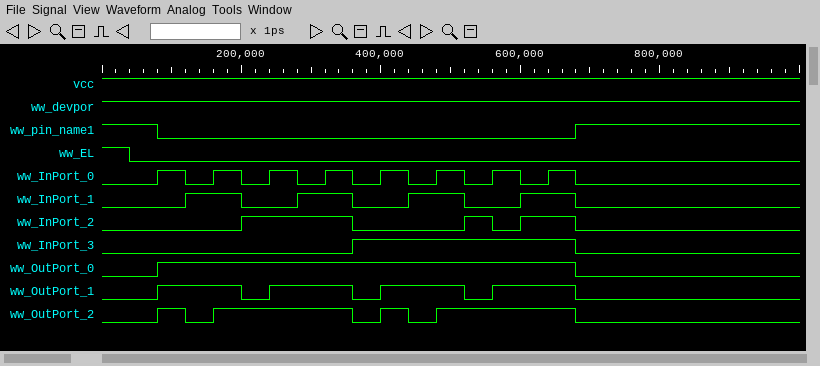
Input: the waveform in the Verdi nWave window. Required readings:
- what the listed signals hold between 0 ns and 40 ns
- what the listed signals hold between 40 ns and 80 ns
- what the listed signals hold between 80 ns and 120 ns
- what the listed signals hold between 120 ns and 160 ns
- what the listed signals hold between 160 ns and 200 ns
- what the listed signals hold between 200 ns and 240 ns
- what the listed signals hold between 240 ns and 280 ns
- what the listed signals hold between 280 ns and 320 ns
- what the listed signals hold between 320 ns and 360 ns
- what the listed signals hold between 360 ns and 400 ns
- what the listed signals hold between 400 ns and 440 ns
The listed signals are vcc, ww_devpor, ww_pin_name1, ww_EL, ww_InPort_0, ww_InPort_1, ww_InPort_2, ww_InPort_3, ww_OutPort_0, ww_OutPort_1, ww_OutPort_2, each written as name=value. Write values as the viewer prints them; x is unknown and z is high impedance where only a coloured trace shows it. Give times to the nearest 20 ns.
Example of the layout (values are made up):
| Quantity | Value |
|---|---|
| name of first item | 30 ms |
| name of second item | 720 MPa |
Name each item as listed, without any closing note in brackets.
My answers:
| Quantity | Value |
|---|---|
| what the listed signals hold between 0 ns and 40 ns | vcc=1, ww_devpor=1, ww_pin_name1=1, ww_EL=1, ww_InPort_0=0, ww_InPort_1=0, ww_InPort_2=0, ww_InPort_3=0, ww_OutPort_0=0, ww_OutPort_1=0, ww_OutPort_2=0 |
| what the listed signals hold between 40 ns and 80 ns | vcc=1, ww_devpor=1, ww_pin_name1=1, ww_EL=0, ww_InPort_0=0, ww_InPort_1=0, ww_InPort_2=0, ww_InPort_3=0, ww_OutPort_0=0, ww_OutPort_1=0, ww_OutPort_2=0 |
| what the listed signals hold between 80 ns and 120 ns | vcc=1, ww_devpor=1, ww_pin_name1=0, ww_EL=0, ww_InPort_0=1, ww_InPort_1=0, ww_InPort_2=0, ww_InPort_3=0, ww_OutPort_0=1, ww_OutPort_1=1, ww_OutPort_2=1 |
| what the listed signals hold between 120 ns and 160 ns | vcc=1, ww_devpor=1, ww_pin_name1=0, ww_EL=0, ww_InPort_0=0, ww_InPort_1=1, ww_InPort_2=0, ww_InPort_3=0, ww_OutPort_0=1, ww_OutPort_1=1, ww_OutPort_2=0 |
| what the listed signals hold between 160 ns and 200 ns | vcc=1, ww_devpor=1, ww_pin_name1=0, ww_EL=0, ww_InPort_0=1, ww_InPort_1=1, ww_InPort_2=0, ww_InPort_3=0, ww_OutPort_0=1, ww_OutPort_1=1, ww_OutPort_2=1 |
| what the listed signals hold between 200 ns and 240 ns | vcc=1, ww_devpor=1, ww_pin_name1=0, ww_EL=0, ww_InPort_0=0, ww_InPort_1=0, ww_InPort_2=1, ww_InPort_3=0, ww_OutPort_0=1, ww_OutPort_1=0, ww_OutPort_2=1 |
| what the listed signals hold between 240 ns and 280 ns | vcc=1, ww_devpor=1, ww_pin_name1=0, ww_EL=0, ww_InPort_0=1, ww_InPort_1=0, ww_InPort_2=1, ww_InPort_3=0, ww_OutPort_0=1, ww_OutPort_1=1, ww_OutPort_2=1 |
| what the listed signals hold between 280 ns and 320 ns | vcc=1, ww_devpor=1, ww_pin_name1=0, ww_EL=0, ww_InPort_0=0, ww_InPort_1=1, ww_InPort_2=1, ww_InPort_3=0, ww_OutPort_0=1, ww_OutPort_1=1, ww_OutPort_2=1 |
| what the listed signals hold between 320 ns and 360 ns | vcc=1, ww_devpor=1, ww_pin_name1=0, ww_EL=0, ww_InPort_0=1, ww_InPort_1=1, ww_InPort_2=1, ww_InPort_3=0, ww_OutPort_0=1, ww_OutPort_1=1, ww_OutPort_2=1 |
| what the listed signals hold between 360 ns and 400 ns | vcc=1, ww_devpor=1, ww_pin_name1=0, ww_EL=0, ww_InPort_0=0, ww_InPort_1=0, ww_InPort_2=0, ww_InPort_3=1, ww_OutPort_0=1, ww_OutPort_1=0, ww_OutPort_2=0 |
| what the listed signals hold between 400 ns and 440 ns | vcc=1, ww_devpor=1, ww_pin_name1=0, ww_EL=0, ww_InPort_0=1, ww_InPort_1=0, ww_InPort_2=0, ww_InPort_3=1, ww_OutPort_0=1, ww_OutPort_1=1, ww_OutPort_2=1 |
